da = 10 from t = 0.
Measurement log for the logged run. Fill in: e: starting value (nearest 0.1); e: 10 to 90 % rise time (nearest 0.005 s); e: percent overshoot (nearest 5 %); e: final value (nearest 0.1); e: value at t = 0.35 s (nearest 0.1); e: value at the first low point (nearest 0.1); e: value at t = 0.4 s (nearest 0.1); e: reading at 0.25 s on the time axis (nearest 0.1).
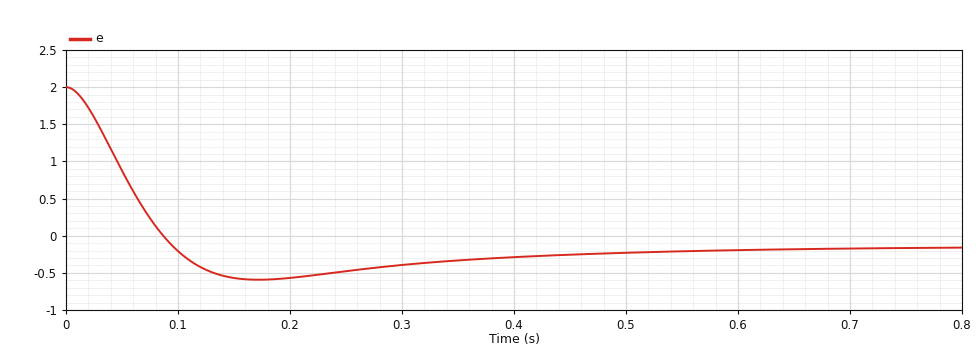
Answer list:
2.0
0.065 s
20 %
-0.2
-0.3
-0.6
-0.3
-0.5
